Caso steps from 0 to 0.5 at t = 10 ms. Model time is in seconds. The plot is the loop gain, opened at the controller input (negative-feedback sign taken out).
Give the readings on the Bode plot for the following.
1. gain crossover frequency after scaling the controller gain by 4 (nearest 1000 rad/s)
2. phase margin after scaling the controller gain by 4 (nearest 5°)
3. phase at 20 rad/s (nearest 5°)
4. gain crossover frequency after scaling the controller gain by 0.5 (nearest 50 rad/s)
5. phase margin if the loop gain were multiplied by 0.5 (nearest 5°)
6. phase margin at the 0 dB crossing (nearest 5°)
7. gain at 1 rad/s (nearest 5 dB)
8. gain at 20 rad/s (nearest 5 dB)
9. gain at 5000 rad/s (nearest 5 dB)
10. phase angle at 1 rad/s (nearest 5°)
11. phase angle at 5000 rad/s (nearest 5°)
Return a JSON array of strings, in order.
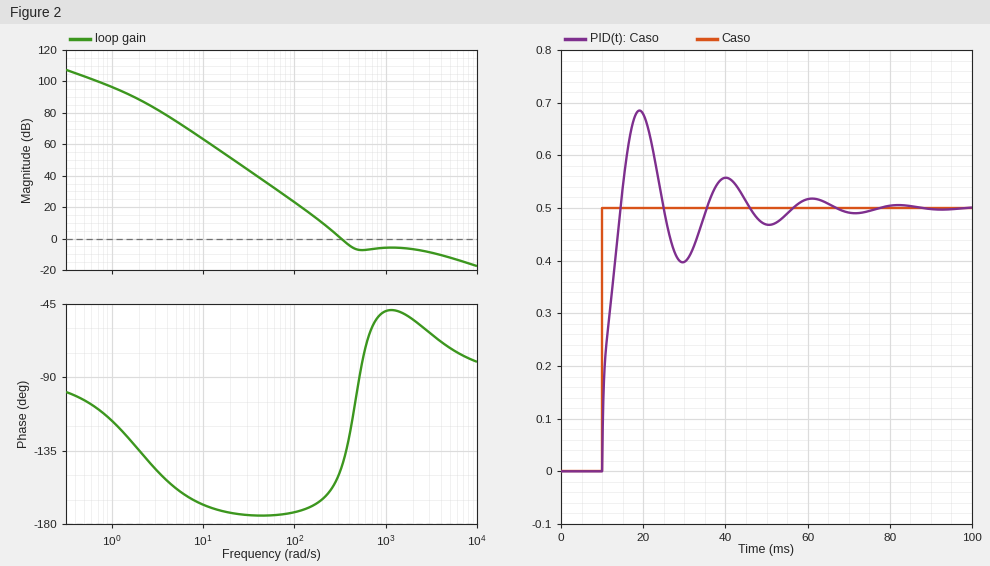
["5000 rad/s", "110°", "-175°", "250 rad/s", "20°", "35°", "95 dB", "50 dB", "-10 dB", "-115°", "-70°"]
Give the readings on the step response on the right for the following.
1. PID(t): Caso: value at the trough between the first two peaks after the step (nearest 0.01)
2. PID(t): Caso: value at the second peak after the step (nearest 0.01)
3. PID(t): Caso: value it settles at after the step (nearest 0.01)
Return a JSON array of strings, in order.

["0.40", "0.56", "0.50"]
